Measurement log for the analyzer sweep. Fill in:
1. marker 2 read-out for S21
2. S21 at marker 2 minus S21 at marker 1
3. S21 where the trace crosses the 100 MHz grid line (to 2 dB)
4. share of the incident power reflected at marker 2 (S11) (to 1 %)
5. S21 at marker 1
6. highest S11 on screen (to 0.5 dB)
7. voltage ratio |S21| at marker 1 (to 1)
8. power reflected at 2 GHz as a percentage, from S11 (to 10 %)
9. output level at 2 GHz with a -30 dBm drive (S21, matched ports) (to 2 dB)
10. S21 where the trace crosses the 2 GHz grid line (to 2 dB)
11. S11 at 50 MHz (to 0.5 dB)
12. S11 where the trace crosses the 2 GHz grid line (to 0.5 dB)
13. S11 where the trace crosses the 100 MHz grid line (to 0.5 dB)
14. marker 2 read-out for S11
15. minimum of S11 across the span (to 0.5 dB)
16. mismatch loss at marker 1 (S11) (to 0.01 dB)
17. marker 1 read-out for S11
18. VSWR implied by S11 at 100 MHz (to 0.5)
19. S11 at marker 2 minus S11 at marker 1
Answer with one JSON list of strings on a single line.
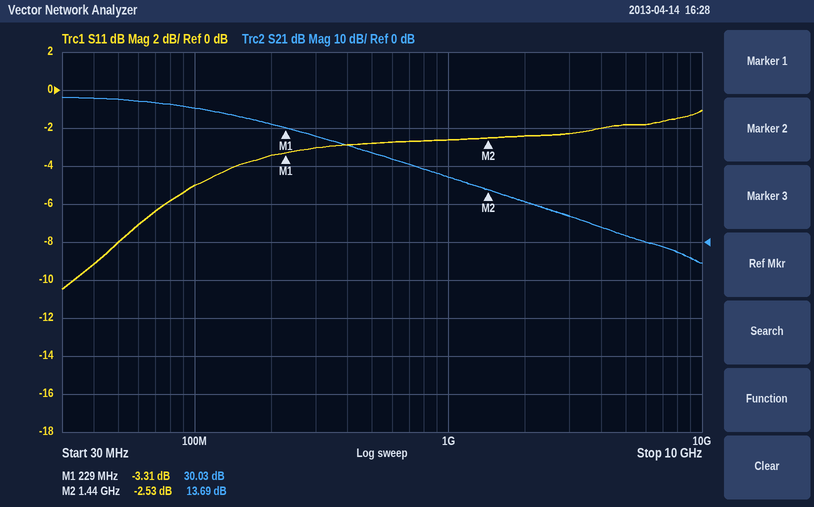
["13.69 dB", "-16.34 dB", "36 dB", "56 %", "30.03 dB", "-1.0 dB", "32", "60 %", "-20 dBm", "10 dB", "-8.0 dB", "-2.5 dB", "-5.0 dB", "-2.53 dB", "-10.5 dB", "2.73 dB", "-3.31 dB", "3.5", "0.78 dB"]
